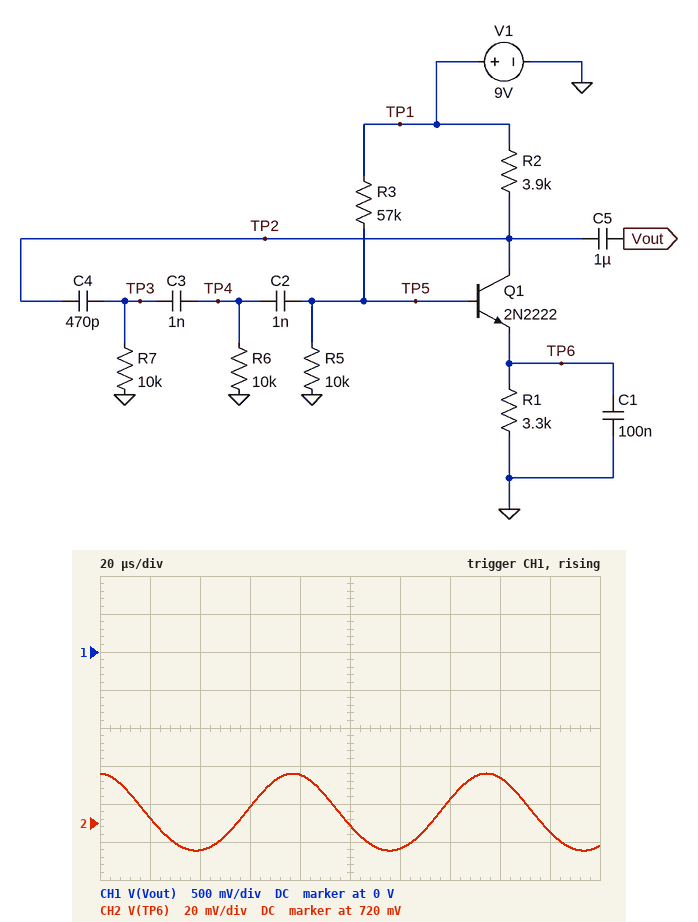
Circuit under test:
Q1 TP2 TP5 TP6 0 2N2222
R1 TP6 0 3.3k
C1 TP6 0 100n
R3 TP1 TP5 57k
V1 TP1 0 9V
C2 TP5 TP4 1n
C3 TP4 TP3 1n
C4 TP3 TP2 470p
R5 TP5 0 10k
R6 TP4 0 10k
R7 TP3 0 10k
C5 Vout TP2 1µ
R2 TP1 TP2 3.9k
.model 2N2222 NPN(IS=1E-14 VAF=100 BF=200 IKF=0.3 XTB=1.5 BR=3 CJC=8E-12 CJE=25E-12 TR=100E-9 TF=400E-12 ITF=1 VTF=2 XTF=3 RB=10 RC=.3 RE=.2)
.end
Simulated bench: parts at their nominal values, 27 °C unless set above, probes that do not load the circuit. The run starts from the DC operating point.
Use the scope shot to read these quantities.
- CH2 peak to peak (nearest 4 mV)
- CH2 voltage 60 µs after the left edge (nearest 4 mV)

40 mV
728 mV
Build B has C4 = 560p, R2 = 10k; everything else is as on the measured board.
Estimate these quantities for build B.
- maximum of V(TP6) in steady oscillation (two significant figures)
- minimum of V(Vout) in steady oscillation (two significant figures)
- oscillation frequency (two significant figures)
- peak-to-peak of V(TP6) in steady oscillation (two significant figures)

790 mV
4.4 V
8.9 kHz
91 mV
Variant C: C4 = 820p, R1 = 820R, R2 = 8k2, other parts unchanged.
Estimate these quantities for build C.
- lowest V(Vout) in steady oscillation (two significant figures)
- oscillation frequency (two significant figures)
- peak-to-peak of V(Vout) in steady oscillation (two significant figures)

670 mV
8.7 kHz
4.4 V
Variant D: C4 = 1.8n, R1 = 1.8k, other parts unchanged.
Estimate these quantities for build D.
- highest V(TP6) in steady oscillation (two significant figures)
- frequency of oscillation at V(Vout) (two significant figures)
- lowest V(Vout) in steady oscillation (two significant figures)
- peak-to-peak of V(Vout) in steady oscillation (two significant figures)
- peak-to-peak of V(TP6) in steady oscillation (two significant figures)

820 mV
8.5 kHz
5.7 V
3.1 V
180 mV
